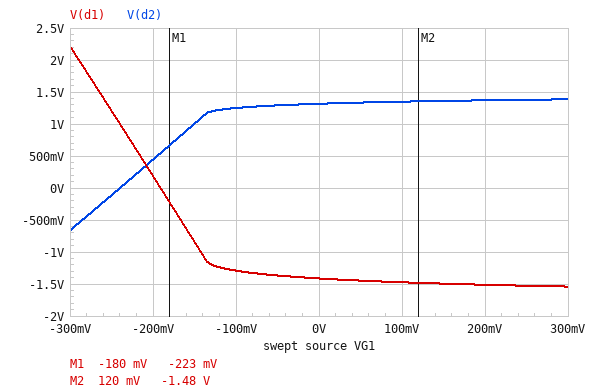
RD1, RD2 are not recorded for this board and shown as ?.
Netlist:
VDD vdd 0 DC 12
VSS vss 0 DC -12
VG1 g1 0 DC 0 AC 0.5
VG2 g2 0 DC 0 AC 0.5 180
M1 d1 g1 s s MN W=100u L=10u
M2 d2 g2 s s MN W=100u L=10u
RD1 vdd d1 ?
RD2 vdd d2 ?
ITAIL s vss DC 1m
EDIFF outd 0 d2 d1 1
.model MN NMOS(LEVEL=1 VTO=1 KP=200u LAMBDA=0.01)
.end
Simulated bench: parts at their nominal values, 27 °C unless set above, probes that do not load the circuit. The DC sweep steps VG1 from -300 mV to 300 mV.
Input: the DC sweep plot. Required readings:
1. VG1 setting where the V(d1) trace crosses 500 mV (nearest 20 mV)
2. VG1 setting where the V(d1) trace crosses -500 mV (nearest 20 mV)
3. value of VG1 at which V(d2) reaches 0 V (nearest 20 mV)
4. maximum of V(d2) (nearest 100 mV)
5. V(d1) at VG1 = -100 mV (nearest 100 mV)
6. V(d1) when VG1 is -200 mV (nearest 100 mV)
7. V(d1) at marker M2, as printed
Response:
-220 mV
-160 mV
-240 mV
1.4 V
-1.3 V
200 mV
-1.48 V
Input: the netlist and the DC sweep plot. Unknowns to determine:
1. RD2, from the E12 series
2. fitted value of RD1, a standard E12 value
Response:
18 kΩ
33 kΩ
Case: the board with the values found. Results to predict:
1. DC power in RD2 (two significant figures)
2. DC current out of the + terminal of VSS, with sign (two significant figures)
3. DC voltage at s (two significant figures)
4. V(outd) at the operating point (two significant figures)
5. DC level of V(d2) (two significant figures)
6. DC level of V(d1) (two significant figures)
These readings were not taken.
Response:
6.3 mW
-1.0 mA
-1.8 V
2.7 V
1.3 V
-1.4 V
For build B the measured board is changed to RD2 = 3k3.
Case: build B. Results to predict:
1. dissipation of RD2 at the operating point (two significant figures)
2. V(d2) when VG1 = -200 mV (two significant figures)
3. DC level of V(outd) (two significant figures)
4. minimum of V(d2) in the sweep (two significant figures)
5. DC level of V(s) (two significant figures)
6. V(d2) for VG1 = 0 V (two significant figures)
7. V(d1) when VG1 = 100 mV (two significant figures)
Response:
1.2 mW
9.8 V
11 V
9.6 V
-1.7 V
10 V
-1.4 V
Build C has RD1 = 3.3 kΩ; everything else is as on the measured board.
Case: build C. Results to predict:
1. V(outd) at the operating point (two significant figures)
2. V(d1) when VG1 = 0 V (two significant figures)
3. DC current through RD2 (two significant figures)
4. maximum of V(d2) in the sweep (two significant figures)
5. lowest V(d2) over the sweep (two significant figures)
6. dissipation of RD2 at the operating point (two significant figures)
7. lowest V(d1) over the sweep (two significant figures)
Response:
-7.0 V
10 V
480 µA
7.0 V
-410 mV
4.2 mW
9.6 V
